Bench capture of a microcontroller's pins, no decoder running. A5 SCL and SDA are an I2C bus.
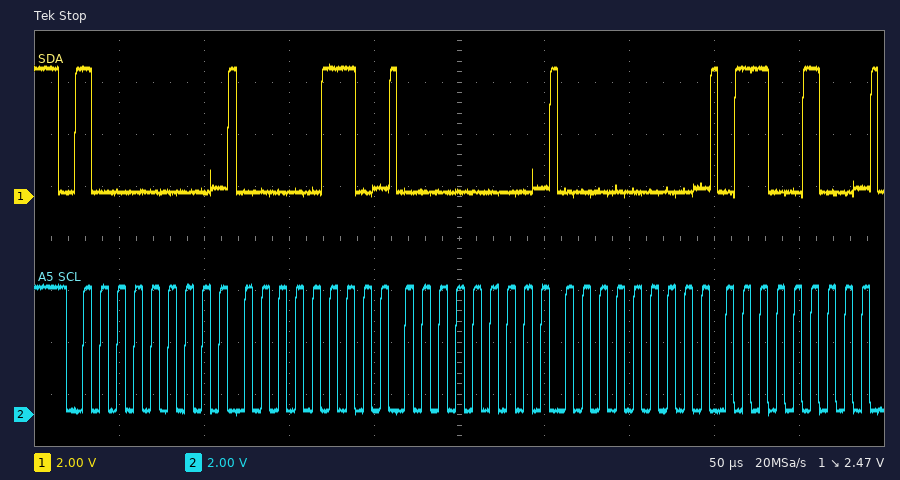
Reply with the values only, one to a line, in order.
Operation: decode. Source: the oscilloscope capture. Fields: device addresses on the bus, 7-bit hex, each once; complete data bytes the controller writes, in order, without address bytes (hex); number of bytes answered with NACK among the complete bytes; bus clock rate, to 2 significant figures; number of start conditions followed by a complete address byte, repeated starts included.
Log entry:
0x40
06 00 00 64
0
100 kHz
1
